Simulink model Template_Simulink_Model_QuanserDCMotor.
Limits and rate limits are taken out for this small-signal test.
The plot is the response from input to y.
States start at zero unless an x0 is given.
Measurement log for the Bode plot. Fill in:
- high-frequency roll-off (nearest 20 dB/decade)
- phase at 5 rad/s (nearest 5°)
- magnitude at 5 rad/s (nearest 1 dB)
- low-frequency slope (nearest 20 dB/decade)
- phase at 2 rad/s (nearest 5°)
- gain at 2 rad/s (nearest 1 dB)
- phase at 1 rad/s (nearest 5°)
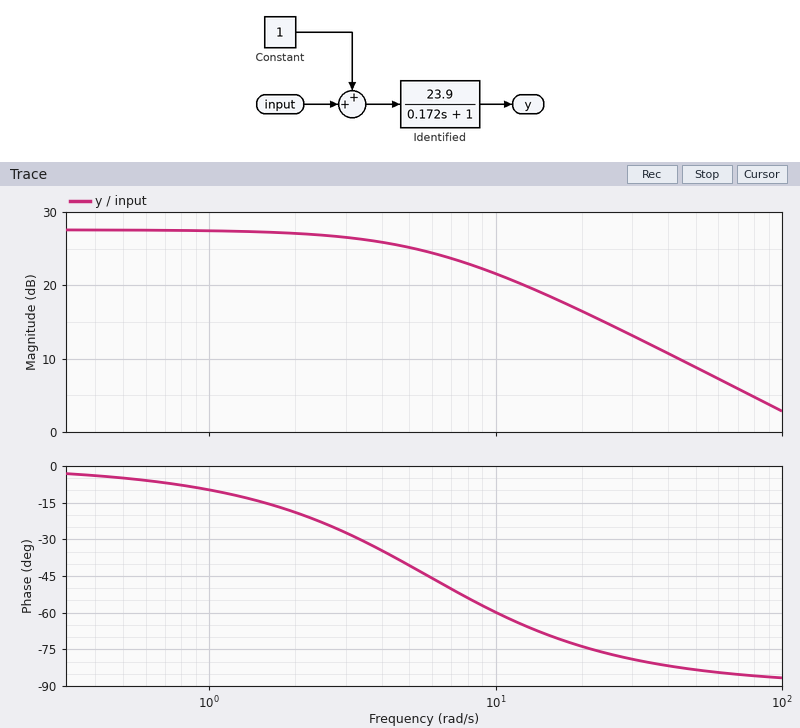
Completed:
-20 dB/decade
-40°
25 dB
0 dB/decade
-20°
27 dB
-10°
